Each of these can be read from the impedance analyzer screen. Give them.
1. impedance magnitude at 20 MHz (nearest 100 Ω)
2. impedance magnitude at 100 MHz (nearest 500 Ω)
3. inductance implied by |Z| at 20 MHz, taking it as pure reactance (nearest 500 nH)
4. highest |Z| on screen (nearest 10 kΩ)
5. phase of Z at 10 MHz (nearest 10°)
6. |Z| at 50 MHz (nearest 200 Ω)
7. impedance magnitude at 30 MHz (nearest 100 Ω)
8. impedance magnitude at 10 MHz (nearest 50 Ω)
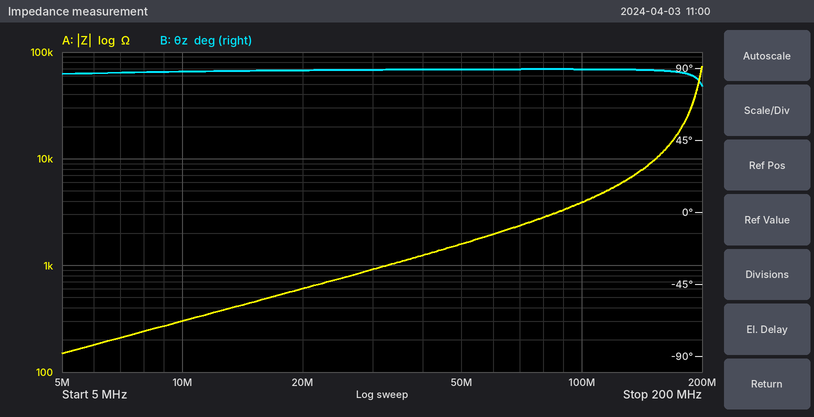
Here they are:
600 Ω
4.0 kΩ
5.0 µH
70 kΩ
90°
1.6 kΩ
900 Ω
300 Ω
